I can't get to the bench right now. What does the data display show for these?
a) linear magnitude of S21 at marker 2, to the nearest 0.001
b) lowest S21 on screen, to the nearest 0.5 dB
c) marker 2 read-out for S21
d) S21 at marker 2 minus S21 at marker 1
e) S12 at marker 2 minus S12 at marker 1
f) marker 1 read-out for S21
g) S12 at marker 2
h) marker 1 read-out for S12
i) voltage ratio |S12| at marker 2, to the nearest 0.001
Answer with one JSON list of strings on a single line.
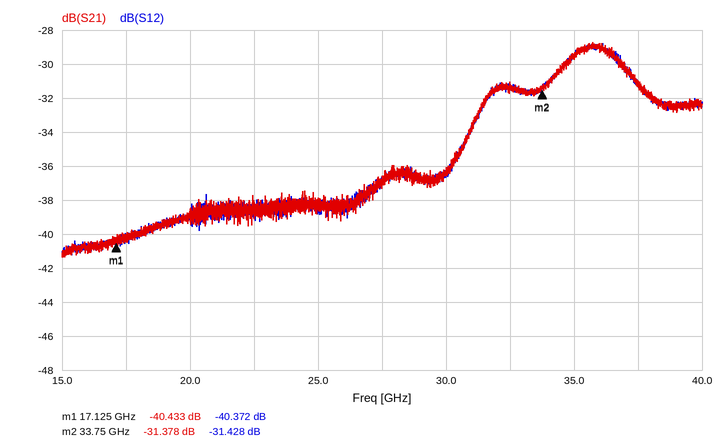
["0.027", "-41.5 dB", "-31.378 dB", "9.055 dB", "8.944 dB", "-40.433 dB", "-31.428 dB", "-40.372 dB", "0.027"]
